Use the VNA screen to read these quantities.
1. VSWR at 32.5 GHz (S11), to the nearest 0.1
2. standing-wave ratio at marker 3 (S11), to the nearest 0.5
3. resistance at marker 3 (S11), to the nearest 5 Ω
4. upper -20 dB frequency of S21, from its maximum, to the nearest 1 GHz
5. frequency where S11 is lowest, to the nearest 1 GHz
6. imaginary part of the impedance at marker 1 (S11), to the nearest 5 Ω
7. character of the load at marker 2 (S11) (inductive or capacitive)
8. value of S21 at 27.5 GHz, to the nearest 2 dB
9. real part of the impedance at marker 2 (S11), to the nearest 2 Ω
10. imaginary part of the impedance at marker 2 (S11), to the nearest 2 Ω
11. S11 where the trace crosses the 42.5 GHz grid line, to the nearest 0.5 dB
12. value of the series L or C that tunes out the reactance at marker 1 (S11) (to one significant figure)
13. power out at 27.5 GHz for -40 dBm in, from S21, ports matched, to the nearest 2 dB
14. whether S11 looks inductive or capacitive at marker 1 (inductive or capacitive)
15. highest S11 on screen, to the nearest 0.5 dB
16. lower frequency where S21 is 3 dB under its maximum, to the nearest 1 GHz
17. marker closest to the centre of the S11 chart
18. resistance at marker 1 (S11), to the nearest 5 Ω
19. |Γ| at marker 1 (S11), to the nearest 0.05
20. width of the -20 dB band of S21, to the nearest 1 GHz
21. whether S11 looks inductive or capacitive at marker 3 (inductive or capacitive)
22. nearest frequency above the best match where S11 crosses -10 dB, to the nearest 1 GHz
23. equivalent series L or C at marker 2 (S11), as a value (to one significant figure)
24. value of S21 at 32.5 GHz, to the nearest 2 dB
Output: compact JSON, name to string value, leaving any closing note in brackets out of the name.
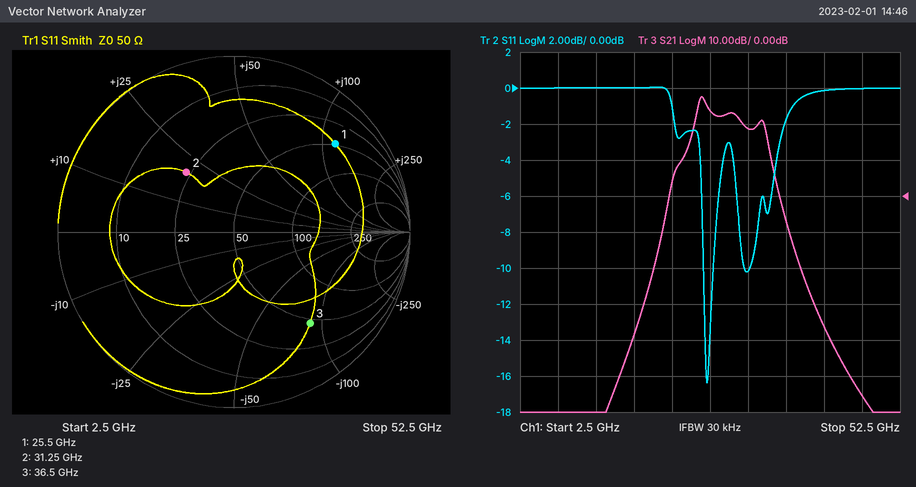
{"VSWR at 32.5 GHz (S11), to the nearest 0.1": "1.9", "standing-wave ratio at marker 3 (S11), to the nearest 0.5": "5.0", "resistance at marker 3 (S11), to the nearest 5 Ω": "45 Ω", "upper -20 dB frequency of S21, from its maximum, to the nearest 1 GHz": "36 GHz", "frequency where S11 is lowest, to the nearest 1 GHz": "27 GHz", "imaginary part of the impedance at marker 1 (S11), to the nearest 5 Ω": "+115 Ω", "character of the load at marker 2 (S11)": "inductive", "value of S21 at 27.5 GHz, to the nearest 2 dB": "24 dB", "real part of the impedance at marker 2 (S11), to the nearest 2 Ω": "24 Ω", "imaginary part of the impedance at marker 2 (S11), to the nearest 2 Ω": "+20 Ω", "S11 where the trace crosses the 42.5 GHz grid line, to the nearest 0.5 dB": "0.0 dB", "value of the series L or C that tunes out the reactance at marker 1 (S11)": "50 fF", "power out at 27.5 GHz for -40 dBm in, from S21, ports matched, to the nearest 2 dB": "-16 dBm", "whether S11 looks inductive or capacitive at marker 1": "inductive", "highest S11 on screen, to the nearest 0.5 dB": "0.0 dB", "lower frequency where S21 is 3 dB under its maximum, to the nearest 1 GHz": "26 GHz", "marker closest to the centre of the S11 chart": "marker 2", "resistance at marker 1 (S11), to the nearest 5 Ω": "50 Ω", "|Γ| at marker 1 (S11), to the nearest 0.05": "0.75", "width of the -20 dB band of S21, to the nearest 1 GHz": "13 GHz", "whether S11 looks inductive or capacitive at marker 3": "capacitive", "nearest frequency above the best match where S11 crosses -10 dB, to the nearest 1 GHz": "28 GHz", "equivalent series L or C at marker 2 (S11), as a value": "100 pH", "value of S21 at 32.5 GHz, to the nearest 2 dB": "18 dB"}
